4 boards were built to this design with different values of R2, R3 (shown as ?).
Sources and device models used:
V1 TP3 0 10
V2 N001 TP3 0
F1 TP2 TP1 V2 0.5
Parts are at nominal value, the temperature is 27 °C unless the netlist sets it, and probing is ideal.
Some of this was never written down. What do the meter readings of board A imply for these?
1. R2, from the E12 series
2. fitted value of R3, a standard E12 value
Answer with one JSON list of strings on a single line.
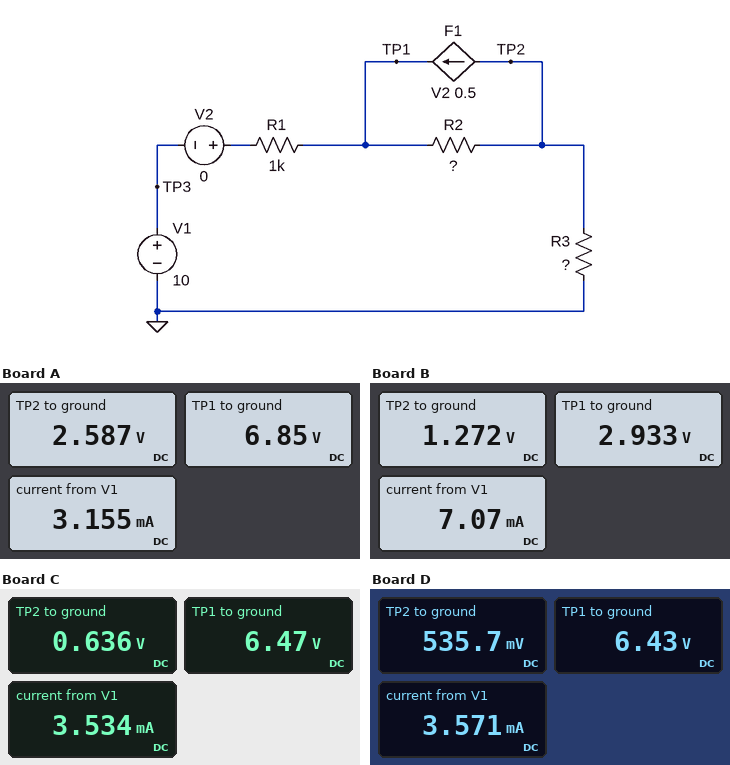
["2.7 kΩ", "820 Ω"]
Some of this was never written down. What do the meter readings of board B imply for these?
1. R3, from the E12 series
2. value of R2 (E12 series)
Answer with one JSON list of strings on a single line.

["180 Ω", "470 Ω"]
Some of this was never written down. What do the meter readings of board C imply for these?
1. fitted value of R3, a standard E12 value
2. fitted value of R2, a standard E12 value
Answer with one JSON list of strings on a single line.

["180 Ω", "3.3 kΩ"]
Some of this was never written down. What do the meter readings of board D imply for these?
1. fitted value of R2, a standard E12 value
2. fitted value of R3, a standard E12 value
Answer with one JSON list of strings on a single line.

["3.3 kΩ", "150 Ω"]
